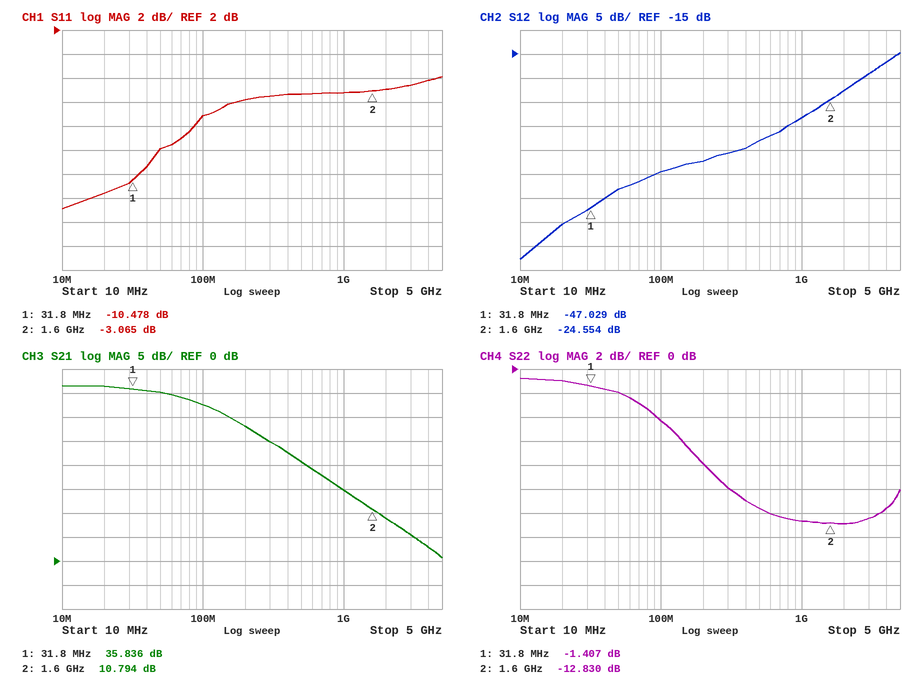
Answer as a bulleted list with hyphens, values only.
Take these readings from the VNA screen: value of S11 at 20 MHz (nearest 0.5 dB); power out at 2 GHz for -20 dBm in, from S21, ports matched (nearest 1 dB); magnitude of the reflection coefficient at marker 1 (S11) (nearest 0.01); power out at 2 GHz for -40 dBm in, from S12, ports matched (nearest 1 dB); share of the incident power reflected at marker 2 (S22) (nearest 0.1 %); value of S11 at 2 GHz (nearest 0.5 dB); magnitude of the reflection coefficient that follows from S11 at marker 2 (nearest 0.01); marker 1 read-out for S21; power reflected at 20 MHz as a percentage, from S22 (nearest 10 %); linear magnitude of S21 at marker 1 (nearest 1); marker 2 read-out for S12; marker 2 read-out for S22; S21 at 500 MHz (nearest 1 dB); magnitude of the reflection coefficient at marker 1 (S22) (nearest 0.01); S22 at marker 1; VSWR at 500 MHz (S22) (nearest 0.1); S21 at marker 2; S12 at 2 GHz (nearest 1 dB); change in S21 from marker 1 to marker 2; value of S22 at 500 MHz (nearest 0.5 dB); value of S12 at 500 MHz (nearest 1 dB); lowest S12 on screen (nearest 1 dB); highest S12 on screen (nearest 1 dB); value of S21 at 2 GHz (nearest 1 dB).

- -11.5 dB
- -11 dBm
- 0.30
- -63 dBm
- 5.2 %
- -3.0 dB
- 0.70
- 35.836 dB
- 80 %
- 62
- -24.554 dB
- -12.830 dB
- 21 dB
- 0.85
- -1.407 dB
- 1.7
- 10.794 dB
- -23 dB
- -25.042 dB
- -11.5 dB
- -33 dB
- -58 dB
- -15 dB
- 9 dB
